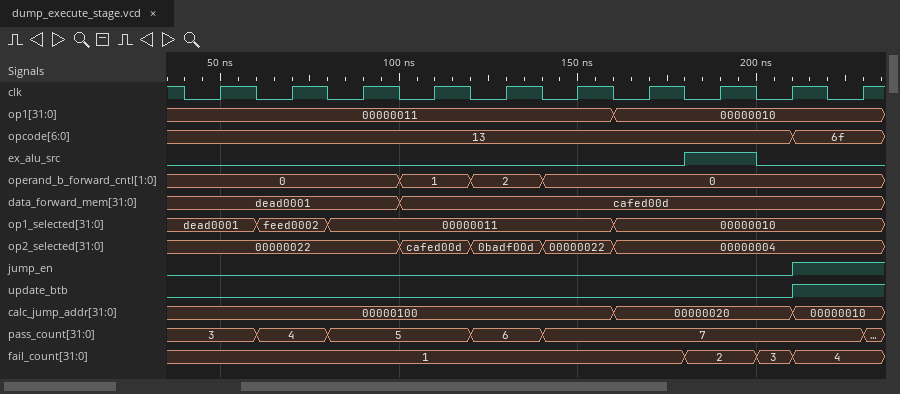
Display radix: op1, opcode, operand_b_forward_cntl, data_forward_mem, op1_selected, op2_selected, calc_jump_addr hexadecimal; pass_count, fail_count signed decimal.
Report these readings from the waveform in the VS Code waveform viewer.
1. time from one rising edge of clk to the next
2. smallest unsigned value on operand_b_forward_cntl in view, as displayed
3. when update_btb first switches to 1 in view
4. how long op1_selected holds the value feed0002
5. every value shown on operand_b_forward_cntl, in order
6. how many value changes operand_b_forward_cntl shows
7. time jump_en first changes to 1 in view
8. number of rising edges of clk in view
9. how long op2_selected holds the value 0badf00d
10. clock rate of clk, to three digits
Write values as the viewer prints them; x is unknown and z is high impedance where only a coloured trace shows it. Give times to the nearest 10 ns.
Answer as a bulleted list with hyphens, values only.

- 20 ns
- 0
- 210 ns
- 20 ns
- 0, 1, 2, 0
- 3
- 210 ns
- 10
- 20 ns
- 50.0 MHz
